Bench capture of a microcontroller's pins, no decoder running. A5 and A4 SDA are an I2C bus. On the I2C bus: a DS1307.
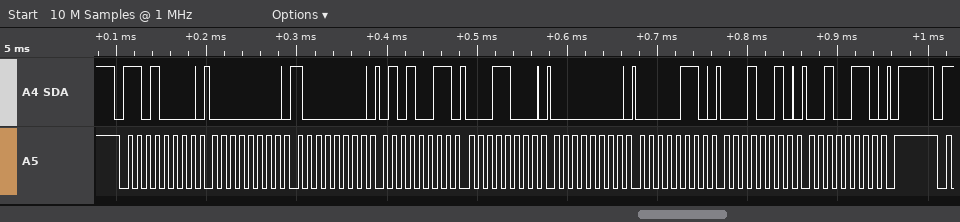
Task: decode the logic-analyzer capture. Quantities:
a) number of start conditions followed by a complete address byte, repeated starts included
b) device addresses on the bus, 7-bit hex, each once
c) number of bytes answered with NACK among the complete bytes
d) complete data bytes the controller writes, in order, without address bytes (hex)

1
0x68
0
00 80 53 18 00 06 12 26
